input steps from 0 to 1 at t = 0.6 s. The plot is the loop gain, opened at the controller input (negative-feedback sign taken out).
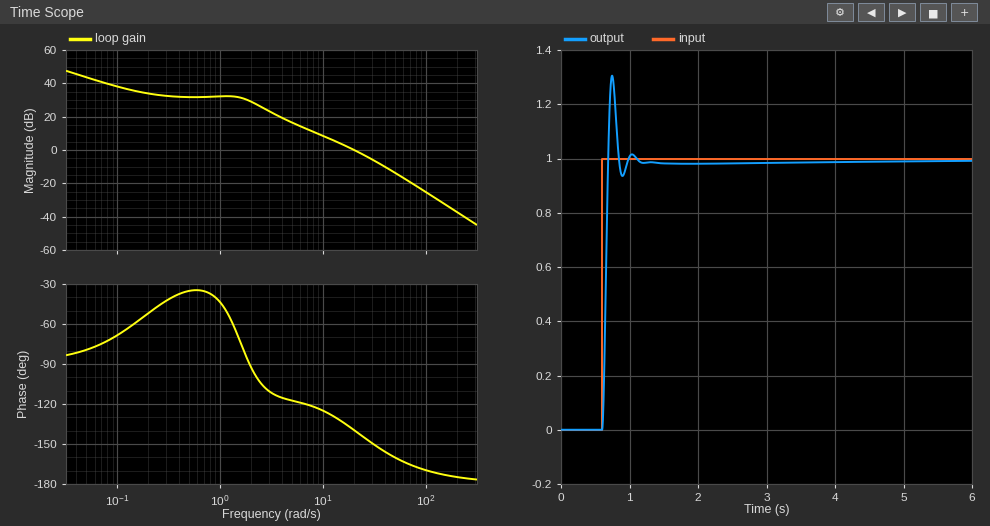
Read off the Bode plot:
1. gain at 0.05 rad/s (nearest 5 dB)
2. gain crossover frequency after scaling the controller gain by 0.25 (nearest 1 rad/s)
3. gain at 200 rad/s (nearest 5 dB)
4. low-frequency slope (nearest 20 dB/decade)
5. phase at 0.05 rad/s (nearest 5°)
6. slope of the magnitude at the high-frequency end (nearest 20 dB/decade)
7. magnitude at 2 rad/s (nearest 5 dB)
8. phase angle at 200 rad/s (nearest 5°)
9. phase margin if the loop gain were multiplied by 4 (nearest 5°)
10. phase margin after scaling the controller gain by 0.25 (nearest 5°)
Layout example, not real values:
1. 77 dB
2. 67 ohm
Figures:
1. 45 dB
2. 7 rad/s
3. -35 dB
4. -20 dB/decade
5. -80°
6. -40 dB/decade
7. 30 dB
8. -175°
9. 20°
10. 60°
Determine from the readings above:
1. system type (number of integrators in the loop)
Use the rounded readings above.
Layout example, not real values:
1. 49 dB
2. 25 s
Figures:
1. 1
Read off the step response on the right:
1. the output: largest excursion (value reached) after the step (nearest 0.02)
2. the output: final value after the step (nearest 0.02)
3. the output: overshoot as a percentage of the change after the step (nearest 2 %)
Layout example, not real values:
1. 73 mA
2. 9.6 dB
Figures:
1. 1.30
2. 1.00
3. 30 %
